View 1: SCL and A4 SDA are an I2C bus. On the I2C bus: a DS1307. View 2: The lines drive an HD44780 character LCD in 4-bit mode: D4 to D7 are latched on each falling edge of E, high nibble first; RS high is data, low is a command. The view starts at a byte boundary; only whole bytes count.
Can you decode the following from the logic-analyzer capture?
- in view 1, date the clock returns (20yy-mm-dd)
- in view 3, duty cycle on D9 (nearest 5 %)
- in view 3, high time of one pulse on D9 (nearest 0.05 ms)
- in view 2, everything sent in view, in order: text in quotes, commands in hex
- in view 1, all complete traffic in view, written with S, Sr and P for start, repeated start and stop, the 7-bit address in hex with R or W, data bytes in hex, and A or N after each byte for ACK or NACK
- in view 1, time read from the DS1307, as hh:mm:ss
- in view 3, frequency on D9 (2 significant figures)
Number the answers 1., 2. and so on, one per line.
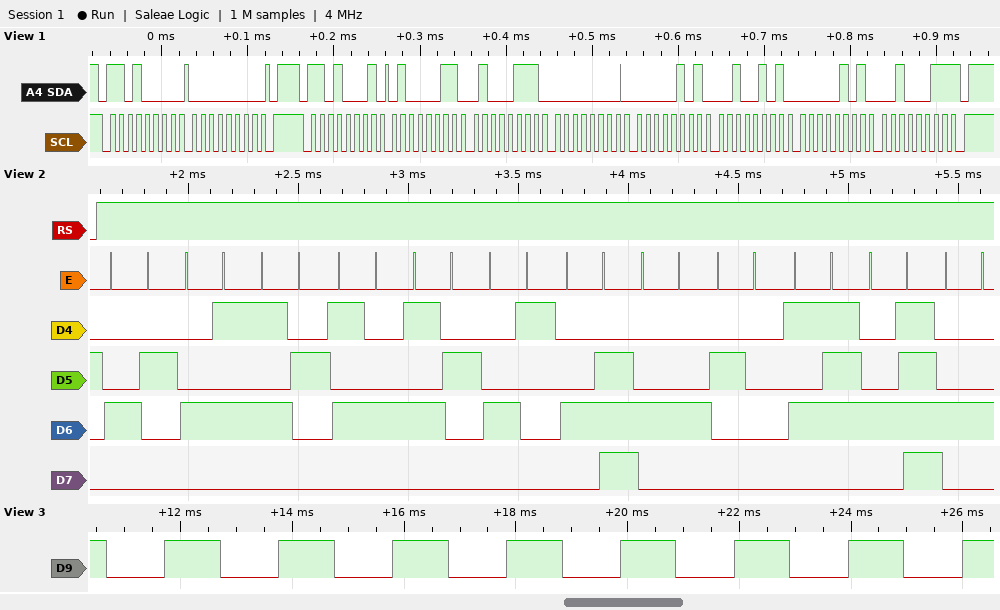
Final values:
1. 2023-05-25
2. 50 %
3. 1.00 ms
4. "BERTRAND WOD"
5. S 68W A 00 A P S 68R A 43 A 47 A 00 A 05 A 25 A 05 A 23 N P
6. 00:47:43
7. 490 Hz
